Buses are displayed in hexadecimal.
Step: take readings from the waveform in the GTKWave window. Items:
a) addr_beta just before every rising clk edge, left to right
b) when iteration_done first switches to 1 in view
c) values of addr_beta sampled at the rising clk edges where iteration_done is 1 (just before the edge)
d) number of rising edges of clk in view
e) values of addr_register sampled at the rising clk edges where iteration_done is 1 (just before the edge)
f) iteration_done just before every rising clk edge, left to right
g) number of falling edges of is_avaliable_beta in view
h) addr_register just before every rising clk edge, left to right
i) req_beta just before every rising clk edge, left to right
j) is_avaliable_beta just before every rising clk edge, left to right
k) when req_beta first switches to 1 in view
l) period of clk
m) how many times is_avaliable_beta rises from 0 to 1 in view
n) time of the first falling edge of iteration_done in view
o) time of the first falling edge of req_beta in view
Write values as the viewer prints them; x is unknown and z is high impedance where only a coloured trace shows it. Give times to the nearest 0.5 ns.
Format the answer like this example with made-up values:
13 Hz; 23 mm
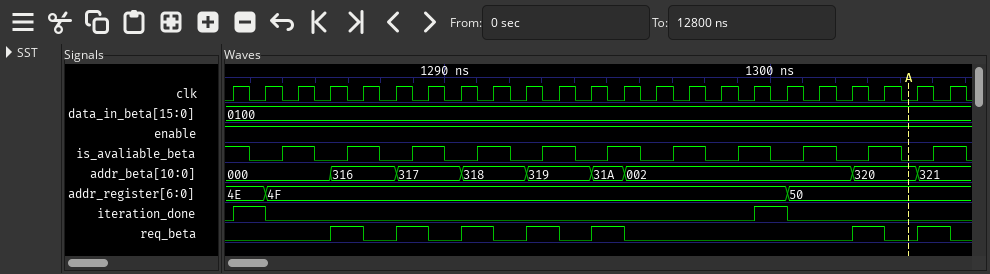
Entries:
000, 000, 000, 000, 316, 316, 317, 317, 318, 318, 319, 319, 31A, 002, 002, 002, 002, 002, 002, 002, 320, 320, 321; 1283.5 ns; 000, 002; 23; 4E, 4F; 0 1 0 0 0 0 0 0 0 0 0 0 0 0 0 0 0 1 0 0 0 0 0; 12; 4E, 4E, 4F, 4F, 4F, 4F, 4F, 4F, 4F, 4F, 4F, 4F, 4F, 4F, 4F, 4F, 4F, 4F, 50, 50, 50, 50, 50; 0 0 0 0 1 0 1 0 1 0 1 0 1 0 0 0 0 0 0 0 1 0 1; 1 0 1 0 1 0 1 0 1 0 1 0 1 0 1 0 1 0 1 0 1 0 1; 1286.5 ns; 1 ns; 11; 1284.5 ns; 1287.5 ns
